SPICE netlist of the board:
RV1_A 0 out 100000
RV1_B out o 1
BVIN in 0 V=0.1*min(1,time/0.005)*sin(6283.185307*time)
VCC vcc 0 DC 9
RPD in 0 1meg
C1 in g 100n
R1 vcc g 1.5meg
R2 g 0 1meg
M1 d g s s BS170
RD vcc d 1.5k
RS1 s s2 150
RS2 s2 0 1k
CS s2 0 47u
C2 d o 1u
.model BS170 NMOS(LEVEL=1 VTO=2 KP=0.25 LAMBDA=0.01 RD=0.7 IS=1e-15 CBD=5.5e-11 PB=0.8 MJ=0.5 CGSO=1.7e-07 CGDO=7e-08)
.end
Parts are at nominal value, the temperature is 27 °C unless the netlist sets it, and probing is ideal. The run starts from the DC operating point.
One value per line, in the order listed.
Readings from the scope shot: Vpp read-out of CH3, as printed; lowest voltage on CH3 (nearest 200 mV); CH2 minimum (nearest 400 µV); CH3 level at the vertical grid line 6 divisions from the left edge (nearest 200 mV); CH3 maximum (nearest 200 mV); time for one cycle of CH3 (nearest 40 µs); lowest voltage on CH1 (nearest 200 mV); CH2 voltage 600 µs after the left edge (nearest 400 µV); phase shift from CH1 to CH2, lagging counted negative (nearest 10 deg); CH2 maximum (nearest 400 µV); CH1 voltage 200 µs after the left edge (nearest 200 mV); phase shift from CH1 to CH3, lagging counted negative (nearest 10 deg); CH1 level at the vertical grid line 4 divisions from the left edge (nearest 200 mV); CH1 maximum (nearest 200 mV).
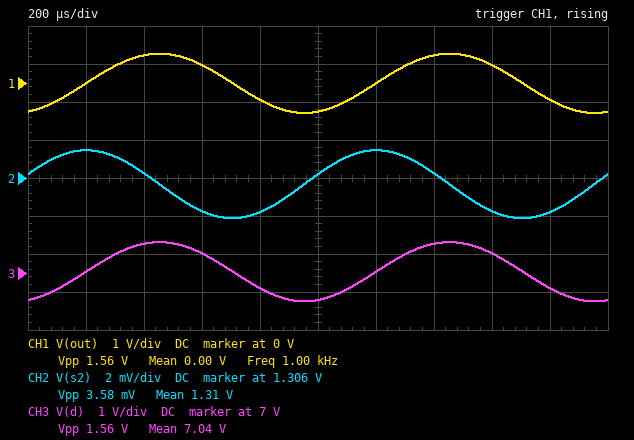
1.56 V
6.2 V
1.3040 V
7.0 V
7.8 V
1.00 ms
-800 mV
1.3044 V
90 deg
1.3076 V
0 V
0 deg
-400 mV
800 mV
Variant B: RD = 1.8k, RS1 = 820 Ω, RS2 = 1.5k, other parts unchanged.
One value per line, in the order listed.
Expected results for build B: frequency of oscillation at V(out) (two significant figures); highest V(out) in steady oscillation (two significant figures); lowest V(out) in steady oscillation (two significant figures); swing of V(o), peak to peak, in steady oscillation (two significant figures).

1.0 kHz
200 mV
-200 mV
400 mV
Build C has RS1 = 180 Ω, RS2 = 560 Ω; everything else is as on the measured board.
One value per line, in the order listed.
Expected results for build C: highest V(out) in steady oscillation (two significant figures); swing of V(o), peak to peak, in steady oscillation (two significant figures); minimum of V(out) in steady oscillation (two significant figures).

690 mV
1.4 V
-700 mV
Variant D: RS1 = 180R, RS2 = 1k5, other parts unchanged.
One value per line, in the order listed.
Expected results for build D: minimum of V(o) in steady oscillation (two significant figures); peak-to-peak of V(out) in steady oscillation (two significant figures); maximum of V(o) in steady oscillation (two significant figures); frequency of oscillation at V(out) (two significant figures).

-660 mV
1.3 V
640 mV
1.0 kHz
